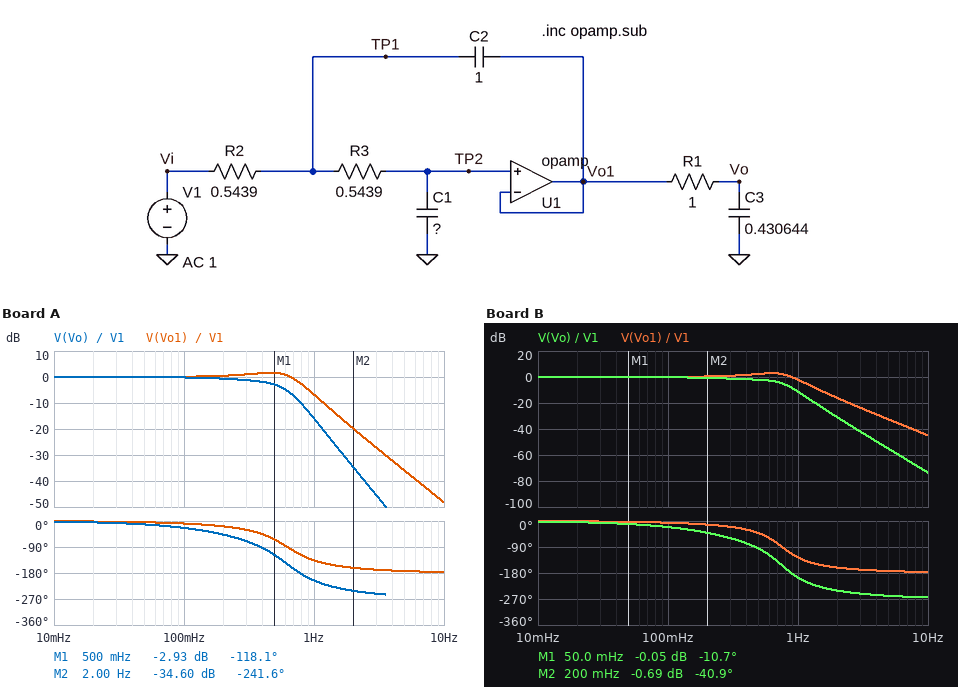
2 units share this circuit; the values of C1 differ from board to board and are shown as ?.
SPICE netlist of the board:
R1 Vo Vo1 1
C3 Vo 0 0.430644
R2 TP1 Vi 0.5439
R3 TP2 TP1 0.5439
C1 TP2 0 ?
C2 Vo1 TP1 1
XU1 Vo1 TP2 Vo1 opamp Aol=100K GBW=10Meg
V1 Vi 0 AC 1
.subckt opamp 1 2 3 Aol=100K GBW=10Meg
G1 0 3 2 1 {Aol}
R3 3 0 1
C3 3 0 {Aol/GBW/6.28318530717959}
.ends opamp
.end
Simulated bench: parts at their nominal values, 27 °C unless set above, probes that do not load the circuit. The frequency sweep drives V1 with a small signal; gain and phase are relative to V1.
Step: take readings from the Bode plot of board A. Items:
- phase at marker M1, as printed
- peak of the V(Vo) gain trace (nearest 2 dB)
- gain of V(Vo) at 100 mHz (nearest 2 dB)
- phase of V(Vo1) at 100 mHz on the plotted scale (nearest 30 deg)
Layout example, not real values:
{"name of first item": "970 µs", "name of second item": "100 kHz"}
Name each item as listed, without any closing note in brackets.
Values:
{"phase at marker M1, as printed": "-118.1 deg", "peak of the V(Vo) gain trace": "0 dB", "gain of V(Vo) at 100 mHz": "0 dB", "phase of V(Vo1) at 100 mHz on the plotted scale": "0 deg"}
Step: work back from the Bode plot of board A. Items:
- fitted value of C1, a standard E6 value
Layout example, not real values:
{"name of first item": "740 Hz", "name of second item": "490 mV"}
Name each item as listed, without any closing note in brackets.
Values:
{"fitted value of C1, a standard E6 value": "220 mF"}
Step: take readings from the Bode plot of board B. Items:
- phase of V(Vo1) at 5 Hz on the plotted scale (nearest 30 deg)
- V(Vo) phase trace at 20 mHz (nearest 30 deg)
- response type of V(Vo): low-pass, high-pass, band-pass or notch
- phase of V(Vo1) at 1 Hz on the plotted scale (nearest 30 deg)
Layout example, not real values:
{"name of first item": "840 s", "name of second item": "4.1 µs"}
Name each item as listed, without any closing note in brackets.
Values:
{"phase of V(Vo1) at 5 Hz on the plotted scale": "-180 deg", "V(Vo) phase trace at 20 mHz": "0 deg", "response type of V(Vo): low-pass, high-pass, band-pass or notch": "low-pass", "phase of V(Vo1) at 1 Hz on the plotted scale": "-120 deg"}
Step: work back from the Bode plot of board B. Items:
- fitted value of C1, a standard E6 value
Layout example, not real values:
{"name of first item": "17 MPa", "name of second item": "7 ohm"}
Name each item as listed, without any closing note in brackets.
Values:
{"fitted value of C1, a standard E6 value": "150 mF"}
